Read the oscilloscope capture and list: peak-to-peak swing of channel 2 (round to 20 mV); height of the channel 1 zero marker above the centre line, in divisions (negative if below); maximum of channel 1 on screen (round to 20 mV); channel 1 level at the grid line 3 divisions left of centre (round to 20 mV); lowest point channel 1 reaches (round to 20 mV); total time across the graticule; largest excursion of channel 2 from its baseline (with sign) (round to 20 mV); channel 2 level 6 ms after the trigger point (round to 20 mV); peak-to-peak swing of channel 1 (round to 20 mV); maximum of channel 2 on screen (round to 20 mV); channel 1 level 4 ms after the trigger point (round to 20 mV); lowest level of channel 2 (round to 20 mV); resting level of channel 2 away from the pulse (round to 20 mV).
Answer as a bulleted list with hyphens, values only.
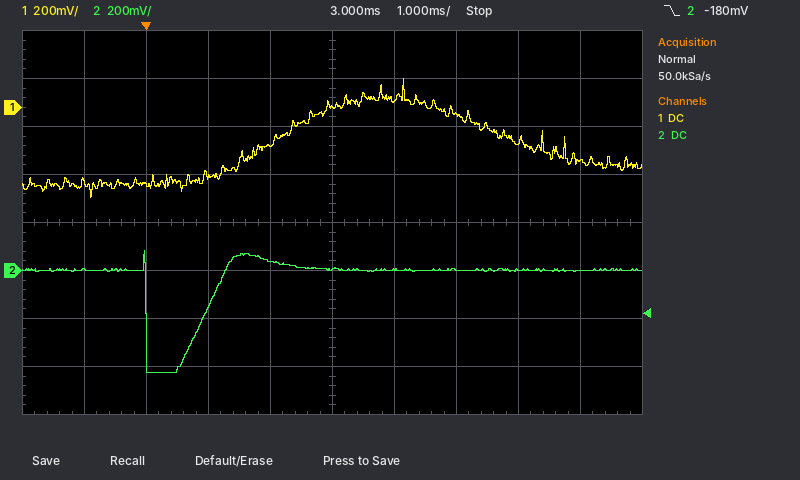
- 500 mV
- +2.4 div
- 120 mV
- -320 mV
- -380 mV
- 10 ms
- -420 mV
- 0 mV
- 500 mV
- 80 mV
- 40 mV
- -420 mV
- 0 mV
